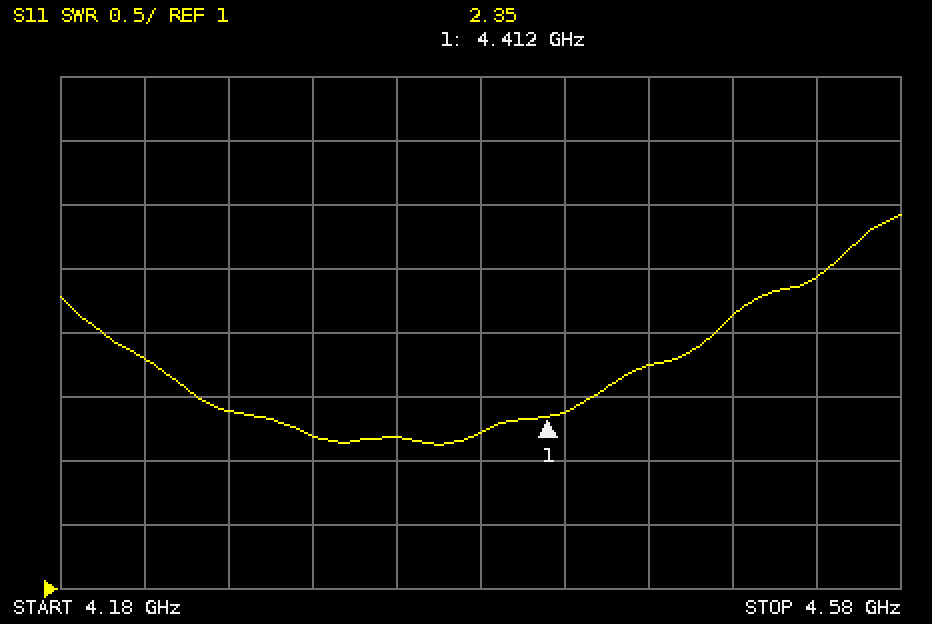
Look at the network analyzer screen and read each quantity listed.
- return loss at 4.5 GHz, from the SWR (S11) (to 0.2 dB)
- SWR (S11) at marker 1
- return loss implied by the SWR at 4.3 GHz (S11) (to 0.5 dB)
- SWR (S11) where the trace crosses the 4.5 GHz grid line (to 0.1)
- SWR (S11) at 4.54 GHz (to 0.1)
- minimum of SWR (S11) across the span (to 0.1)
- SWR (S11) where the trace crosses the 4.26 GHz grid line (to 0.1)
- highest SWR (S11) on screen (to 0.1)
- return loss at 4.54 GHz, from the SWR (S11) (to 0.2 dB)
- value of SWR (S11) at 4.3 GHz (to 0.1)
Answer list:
5.8 dB
2.35
8.5 dB
3.1
3.4
2.1
2.4
3.9
5.2 dB
2.2
